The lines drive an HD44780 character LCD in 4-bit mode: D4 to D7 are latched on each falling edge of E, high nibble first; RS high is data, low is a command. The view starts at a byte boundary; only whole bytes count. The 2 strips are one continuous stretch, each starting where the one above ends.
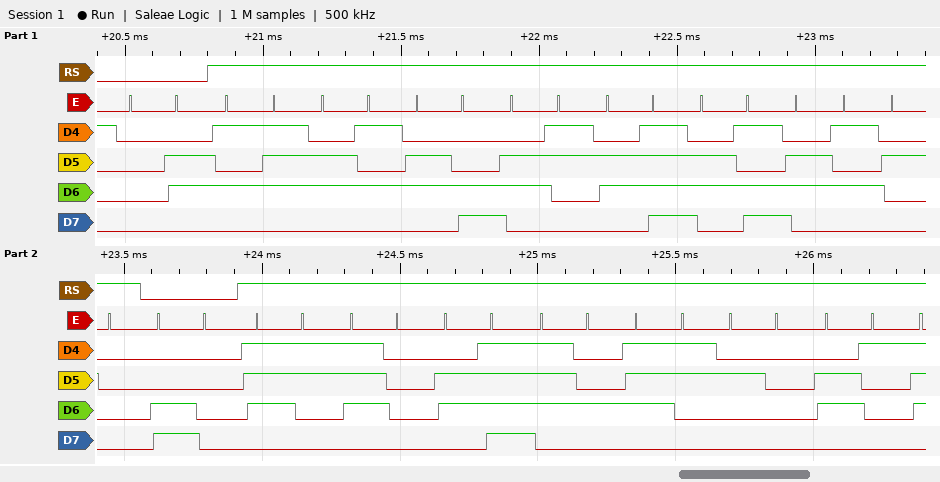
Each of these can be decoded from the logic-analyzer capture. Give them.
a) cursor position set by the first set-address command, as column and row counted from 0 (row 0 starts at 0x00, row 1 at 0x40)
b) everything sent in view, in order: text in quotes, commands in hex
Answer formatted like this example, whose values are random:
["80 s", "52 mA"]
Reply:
["column 0, row 1", "0x06 \"Welcome \" 0xC0 \"spots a\""]
